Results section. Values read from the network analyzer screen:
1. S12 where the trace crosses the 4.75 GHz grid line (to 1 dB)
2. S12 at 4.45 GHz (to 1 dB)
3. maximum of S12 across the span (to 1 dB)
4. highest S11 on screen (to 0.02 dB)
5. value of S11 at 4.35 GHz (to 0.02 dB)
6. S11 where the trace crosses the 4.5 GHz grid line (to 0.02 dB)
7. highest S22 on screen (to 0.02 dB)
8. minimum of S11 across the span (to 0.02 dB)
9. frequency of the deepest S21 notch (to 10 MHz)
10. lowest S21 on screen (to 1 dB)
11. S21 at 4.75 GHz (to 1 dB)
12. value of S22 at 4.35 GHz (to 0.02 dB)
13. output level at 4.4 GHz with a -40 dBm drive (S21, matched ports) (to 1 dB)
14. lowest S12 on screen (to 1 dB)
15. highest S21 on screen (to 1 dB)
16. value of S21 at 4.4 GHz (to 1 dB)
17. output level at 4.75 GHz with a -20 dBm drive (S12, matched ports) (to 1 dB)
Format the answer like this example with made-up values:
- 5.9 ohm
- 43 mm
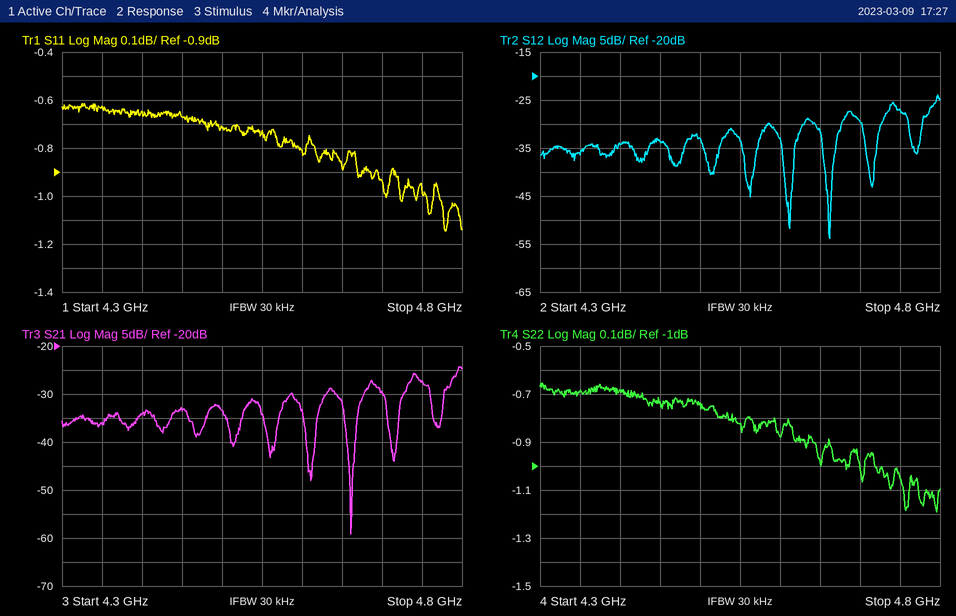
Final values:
- -27 dB
- -34 dB
- -24 dB
- -0.62 dB
- -0.62 dB
- -0.72 dB
- -0.66 dB
- -1.14 dB
- 4.66 GHz
- -59 dB
- -27 dB
- -0.68 dB
- -74 dBm
- -54 dB
- -24 dB
- -34 dB
- -47 dBm
